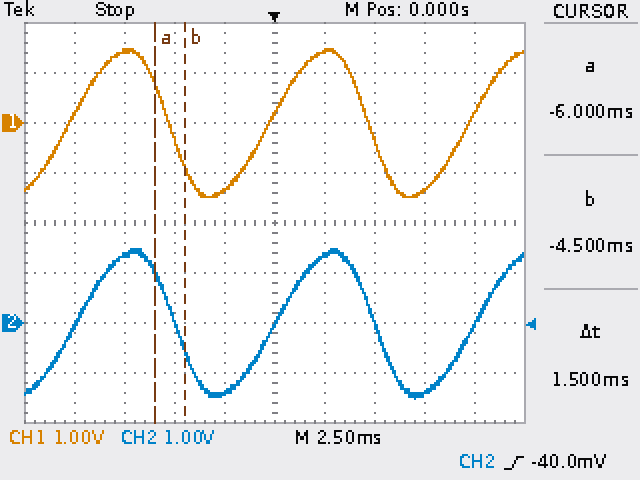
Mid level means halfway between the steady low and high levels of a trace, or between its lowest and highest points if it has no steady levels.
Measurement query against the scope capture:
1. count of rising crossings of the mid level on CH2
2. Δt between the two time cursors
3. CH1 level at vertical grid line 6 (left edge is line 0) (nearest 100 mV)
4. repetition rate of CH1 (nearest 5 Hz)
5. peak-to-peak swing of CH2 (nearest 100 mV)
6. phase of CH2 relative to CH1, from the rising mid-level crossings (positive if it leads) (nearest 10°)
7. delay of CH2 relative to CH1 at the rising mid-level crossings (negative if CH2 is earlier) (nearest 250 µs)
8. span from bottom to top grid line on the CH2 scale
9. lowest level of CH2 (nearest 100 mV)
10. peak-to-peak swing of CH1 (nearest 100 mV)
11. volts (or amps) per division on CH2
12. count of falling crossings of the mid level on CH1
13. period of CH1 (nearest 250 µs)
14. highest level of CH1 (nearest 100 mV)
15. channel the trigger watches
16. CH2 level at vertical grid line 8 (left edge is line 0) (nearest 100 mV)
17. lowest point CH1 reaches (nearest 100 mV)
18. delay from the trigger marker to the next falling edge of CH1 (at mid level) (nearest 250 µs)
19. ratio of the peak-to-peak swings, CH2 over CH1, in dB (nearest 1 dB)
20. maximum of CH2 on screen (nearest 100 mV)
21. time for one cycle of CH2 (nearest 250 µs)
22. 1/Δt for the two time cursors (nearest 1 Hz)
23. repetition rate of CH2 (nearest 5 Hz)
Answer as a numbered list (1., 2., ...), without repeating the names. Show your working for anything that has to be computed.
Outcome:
1. 3
2. 1.5 ms
3. 1.4 V
4. 1 / 10.00 ms ≈ 100 Hz
5. 1.5 V − (-1.5 V) = 3.0 V
6. −360° × (+250 µs) / 10.00 ms ≈ -9.00°, so -10° to the nearest 10°
7. +250 µs
8. 8 V
9. -1.5 V
10. 1.5 V − (-1.5 V) = 3.0 V
11. 1 V
12. 2
13. 10.00 ms
14. 1.5 V
15. CH2
16. -1.4 V
17. -1.5 V
18. 4.75 ms
19. 20 log10(3.0 V / 3.0 V) ≈ 0 dB
20. 1.5 V
21. 10.00 ms
22. 1 / 1.5 ms ≈ 667 Hz
23. 1 / 10.00 ms ≈ 100 Hz
